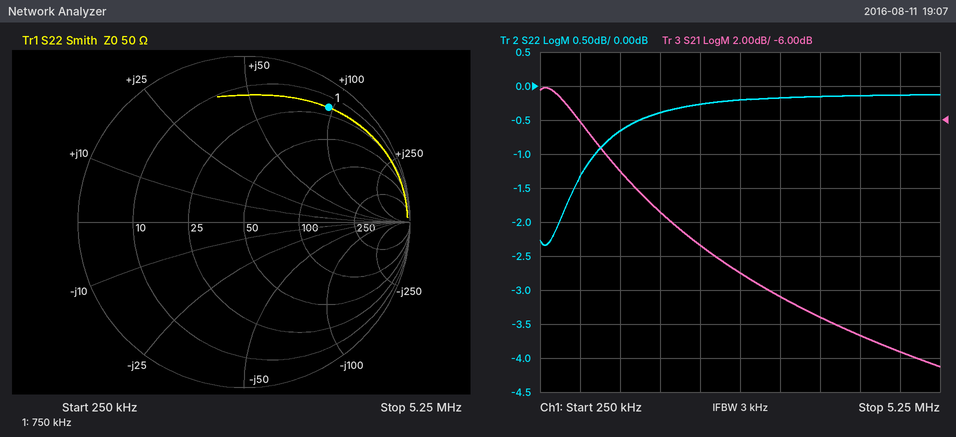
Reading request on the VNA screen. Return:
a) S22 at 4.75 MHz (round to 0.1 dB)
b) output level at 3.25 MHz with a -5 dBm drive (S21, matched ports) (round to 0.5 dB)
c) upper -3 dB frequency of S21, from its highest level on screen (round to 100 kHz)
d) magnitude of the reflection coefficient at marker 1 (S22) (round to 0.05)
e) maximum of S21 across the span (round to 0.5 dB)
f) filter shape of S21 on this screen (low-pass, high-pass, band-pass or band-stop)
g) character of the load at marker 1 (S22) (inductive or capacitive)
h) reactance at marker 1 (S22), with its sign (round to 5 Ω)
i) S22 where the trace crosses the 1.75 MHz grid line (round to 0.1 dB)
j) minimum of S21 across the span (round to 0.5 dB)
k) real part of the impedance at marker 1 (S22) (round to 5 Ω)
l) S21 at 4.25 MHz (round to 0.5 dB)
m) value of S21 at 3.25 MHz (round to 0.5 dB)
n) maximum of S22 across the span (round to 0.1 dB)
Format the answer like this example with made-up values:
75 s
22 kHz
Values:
-0.1 dB
-21.5 dBm
900 kHz
0.85
-4.0 dB
low-pass
inductive
+95 Ω
-0.4 dB
-20.5 dB
20 Ω
-18.5 dB
-16.5 dB
-0.1 dB
